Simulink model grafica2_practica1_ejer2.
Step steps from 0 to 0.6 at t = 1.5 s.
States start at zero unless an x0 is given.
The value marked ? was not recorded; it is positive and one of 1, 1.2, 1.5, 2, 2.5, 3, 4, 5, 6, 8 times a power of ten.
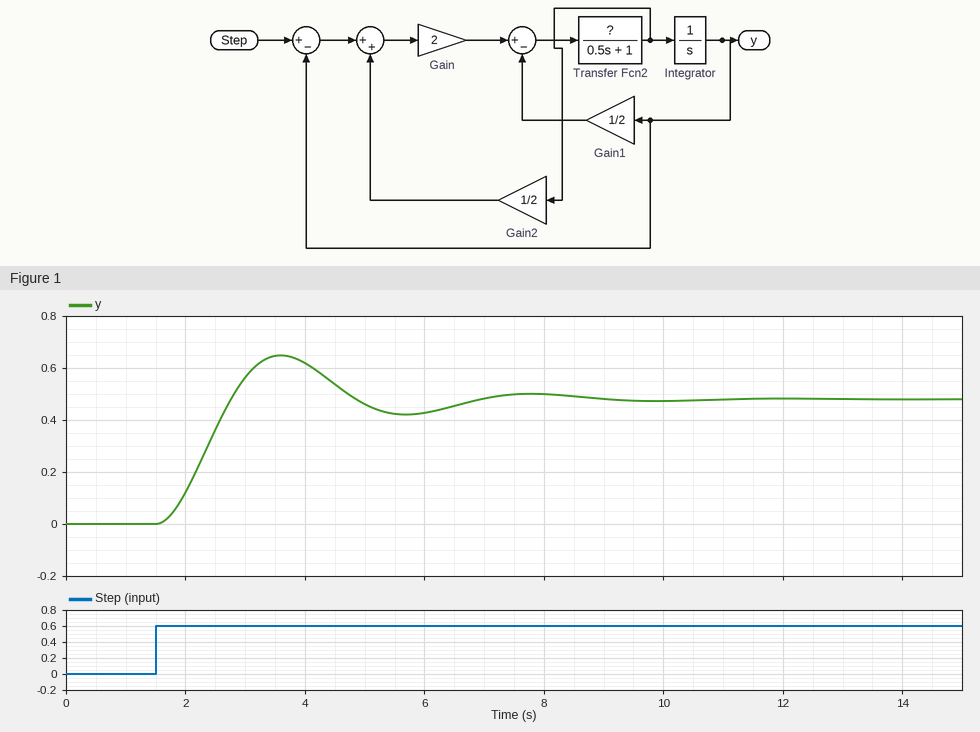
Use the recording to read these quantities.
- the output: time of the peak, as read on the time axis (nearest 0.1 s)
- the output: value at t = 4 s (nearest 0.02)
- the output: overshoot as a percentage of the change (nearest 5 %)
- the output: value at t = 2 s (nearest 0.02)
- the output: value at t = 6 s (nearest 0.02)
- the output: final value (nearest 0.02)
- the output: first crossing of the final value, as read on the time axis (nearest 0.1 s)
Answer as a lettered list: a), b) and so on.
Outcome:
a) 3.6 s
b) 0.62
c) 35 %
d) 0.12
e) 0.42
f) 0.48
g) 2.8 s
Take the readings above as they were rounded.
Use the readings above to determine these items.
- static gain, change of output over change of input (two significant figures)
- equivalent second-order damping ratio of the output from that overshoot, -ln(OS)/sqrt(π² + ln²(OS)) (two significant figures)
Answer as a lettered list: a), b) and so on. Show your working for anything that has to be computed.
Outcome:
a) (0.48 - 0) / (0.6 - 0) = 0.80
b) ln(0.35) = -1.050; 1.050 / sqrt(9.870 + 1.102) = 0.32
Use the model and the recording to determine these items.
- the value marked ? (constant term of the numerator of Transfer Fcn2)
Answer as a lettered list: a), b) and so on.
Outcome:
a) 0.5
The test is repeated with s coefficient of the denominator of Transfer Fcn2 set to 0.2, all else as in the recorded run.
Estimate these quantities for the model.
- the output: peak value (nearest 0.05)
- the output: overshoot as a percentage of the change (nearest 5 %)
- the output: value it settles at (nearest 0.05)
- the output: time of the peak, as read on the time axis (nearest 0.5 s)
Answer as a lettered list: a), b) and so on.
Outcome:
a) 0.55
b) 15 %
c) 0.50
d) 3.0 s
